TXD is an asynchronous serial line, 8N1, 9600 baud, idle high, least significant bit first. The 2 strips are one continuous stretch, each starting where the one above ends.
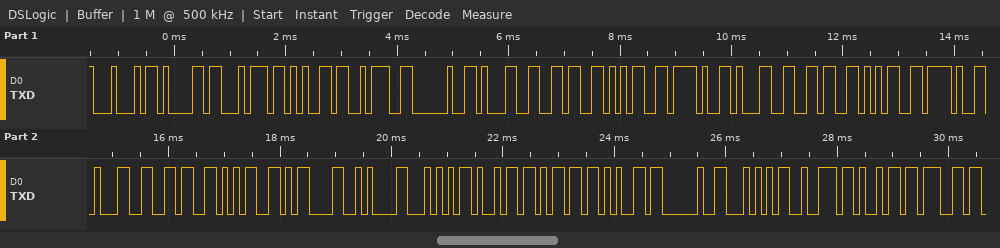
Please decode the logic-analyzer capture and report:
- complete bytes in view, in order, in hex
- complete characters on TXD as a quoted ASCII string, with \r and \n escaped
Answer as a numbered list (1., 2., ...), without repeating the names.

1. 44 61 74 65 3A 20 31 36 35 2F 31 36 35 2F 31 36 35 0D 0A 54 69 6D 65 20 54 72 69 67
2. "Date: 165/165/165\r\nTime Trig"
